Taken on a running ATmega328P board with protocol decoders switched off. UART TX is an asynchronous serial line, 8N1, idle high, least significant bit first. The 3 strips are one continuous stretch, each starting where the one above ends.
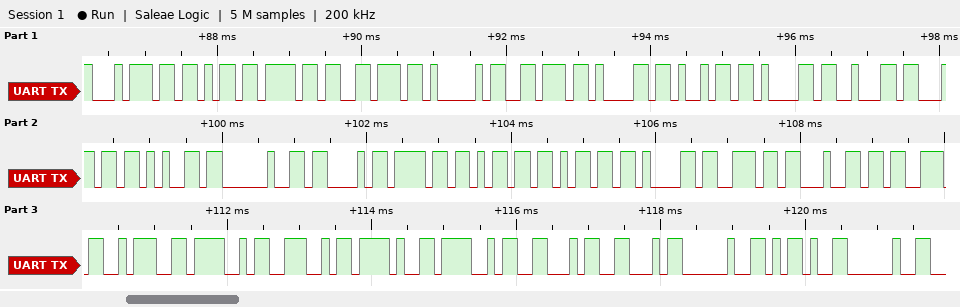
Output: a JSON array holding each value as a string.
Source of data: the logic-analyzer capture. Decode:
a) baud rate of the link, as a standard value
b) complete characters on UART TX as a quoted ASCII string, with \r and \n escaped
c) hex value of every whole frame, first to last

["9600 baud", "\"tkovAvaiable Commands:ON/OFF - \"", "74 6B 6F 76 41 76 61 69 61 62 6C 65 20 43 6F 6D 6D 61 6E 64 73 3A 4F 4E 2F 4F 46 46 20 2D 20"]
